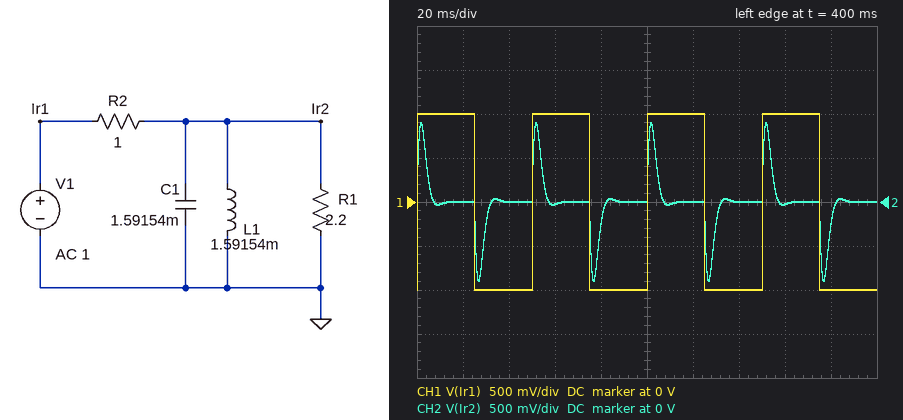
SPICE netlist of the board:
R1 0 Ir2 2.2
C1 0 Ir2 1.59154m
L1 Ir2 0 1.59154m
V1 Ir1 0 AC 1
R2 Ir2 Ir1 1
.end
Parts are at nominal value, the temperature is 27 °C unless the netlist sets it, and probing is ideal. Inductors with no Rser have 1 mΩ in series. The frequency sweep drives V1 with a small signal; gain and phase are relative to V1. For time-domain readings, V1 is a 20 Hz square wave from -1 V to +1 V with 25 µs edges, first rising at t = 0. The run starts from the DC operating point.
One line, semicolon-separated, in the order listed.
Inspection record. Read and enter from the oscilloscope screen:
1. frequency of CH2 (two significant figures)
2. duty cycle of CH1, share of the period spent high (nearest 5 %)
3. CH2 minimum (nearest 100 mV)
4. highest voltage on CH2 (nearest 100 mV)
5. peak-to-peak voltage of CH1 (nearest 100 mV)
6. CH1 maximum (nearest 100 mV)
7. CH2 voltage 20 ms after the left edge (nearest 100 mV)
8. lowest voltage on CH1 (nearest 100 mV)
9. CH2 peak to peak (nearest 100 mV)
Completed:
20 Hz; 50 %; -900 mV; 900 mV; 2.0 V; 1.0 V; 0 V; -1.0 V; 1.8 V
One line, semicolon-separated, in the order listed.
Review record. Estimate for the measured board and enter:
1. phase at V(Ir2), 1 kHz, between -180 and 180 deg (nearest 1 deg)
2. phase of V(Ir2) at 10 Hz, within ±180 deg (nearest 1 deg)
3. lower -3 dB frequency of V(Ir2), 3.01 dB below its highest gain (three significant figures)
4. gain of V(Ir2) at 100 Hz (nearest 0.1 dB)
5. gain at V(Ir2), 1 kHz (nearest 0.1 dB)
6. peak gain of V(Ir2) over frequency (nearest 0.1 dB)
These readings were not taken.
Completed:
-82 deg; 81 deg; 51.0 Hz; -3.3 dB; -20.0 dB; -3.3 dB
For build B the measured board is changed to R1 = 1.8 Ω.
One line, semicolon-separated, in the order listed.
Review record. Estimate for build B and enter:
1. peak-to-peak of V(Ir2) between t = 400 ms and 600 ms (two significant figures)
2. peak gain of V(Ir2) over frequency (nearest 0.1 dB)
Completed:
1.7 V; -3.8 dB
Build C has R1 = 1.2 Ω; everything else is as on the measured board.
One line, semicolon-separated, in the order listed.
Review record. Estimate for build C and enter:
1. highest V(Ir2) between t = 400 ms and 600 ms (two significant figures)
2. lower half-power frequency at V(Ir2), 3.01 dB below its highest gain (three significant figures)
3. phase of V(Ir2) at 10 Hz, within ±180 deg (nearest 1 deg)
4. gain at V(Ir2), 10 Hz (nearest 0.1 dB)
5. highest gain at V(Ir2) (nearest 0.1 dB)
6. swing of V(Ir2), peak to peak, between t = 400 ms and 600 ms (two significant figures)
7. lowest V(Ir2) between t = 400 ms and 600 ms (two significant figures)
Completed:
780 mV; 44.0 Hz; 79 deg; -20.1 dB; -5.3 dB; 1.6 V; -780 mV
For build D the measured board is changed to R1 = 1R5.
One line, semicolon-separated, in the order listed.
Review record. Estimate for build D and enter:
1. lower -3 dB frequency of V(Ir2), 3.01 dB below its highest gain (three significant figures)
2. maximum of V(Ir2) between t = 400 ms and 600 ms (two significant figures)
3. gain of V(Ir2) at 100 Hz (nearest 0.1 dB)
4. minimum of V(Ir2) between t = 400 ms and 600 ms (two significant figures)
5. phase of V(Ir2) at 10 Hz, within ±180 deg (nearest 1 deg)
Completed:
46.9 Hz; 830 mV; -4.4 dB; -830 mV; 80 deg
